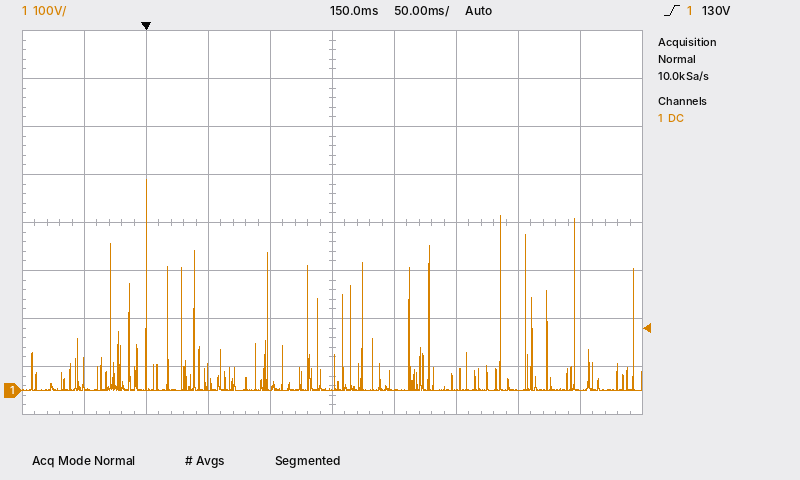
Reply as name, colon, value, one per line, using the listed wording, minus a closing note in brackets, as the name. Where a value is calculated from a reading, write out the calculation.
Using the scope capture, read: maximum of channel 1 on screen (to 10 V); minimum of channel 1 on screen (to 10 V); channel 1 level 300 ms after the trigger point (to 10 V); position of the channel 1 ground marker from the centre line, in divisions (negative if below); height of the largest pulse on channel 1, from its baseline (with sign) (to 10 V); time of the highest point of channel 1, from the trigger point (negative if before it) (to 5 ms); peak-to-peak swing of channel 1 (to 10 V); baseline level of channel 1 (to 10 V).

maximum of channel 1 on screen: 440 V
minimum of channel 1 on screen: 0 V
channel 1 level 300 ms after the trigger point: 0 V
position of the channel 1 ground marker from the centre line, in divisions: -3.5 div
height of the largest pulse on channel 1, from its baseline (with sign): 440 V − (0 V) = +440 V
time of the highest point of channel 1, from the trigger point (negative if before it): 0 ms
peak-to-peak swing of channel 1: 440 V − (0 V) = 440 V
baseline level of channel 1: 0 V
